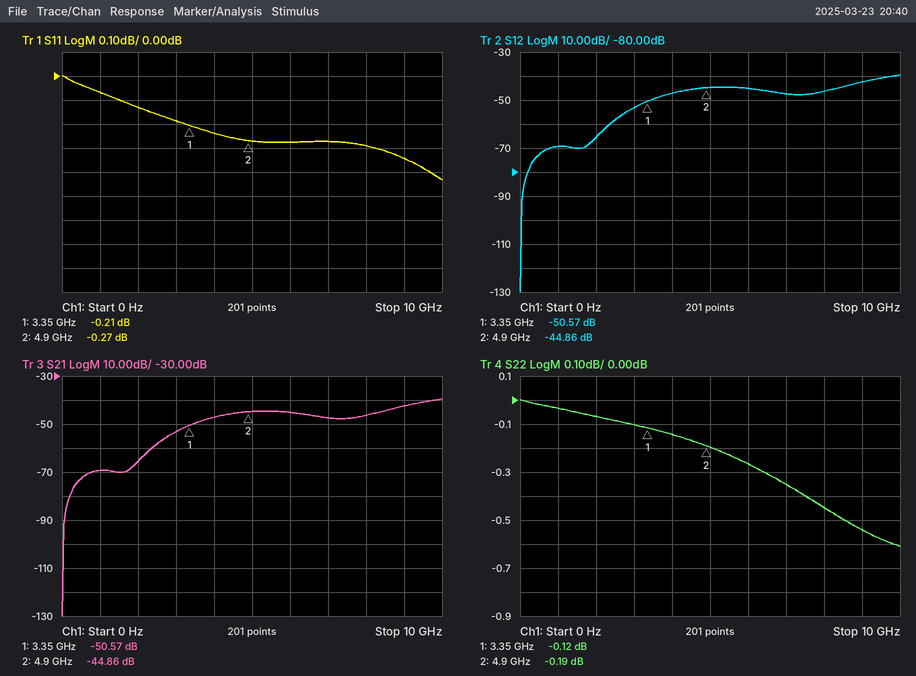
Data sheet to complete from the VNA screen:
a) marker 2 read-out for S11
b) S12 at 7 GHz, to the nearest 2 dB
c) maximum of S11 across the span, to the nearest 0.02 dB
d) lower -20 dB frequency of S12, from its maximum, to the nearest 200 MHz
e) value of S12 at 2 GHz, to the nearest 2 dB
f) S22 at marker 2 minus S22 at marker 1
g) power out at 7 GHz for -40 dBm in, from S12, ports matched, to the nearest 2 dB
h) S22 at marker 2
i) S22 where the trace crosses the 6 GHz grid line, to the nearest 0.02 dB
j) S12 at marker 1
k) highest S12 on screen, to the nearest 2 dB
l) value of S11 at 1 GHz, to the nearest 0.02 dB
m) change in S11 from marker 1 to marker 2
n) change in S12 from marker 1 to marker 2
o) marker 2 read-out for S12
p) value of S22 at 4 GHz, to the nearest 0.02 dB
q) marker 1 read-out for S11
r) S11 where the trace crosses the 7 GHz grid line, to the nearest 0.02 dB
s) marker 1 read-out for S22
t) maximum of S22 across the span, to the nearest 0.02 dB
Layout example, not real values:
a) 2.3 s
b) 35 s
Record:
a) -0.27 dB
b) -48 dB
c) 0.00 dB
d) 2.4 GHz
e) -66 dB
f) -0.07 dB
g) -88 dBm
h) -0.19 dB
i) -0.26 dB
j) -50.57 dB
k) -40 dB
l) -0.06 dB
m) -0.06 dB
n) 5.71 dB
o) -44.86 dB
p) -0.14 dB
q) -0.21 dB
r) -0.28 dB
s) -0.12 dB
t) 0.00 dB
